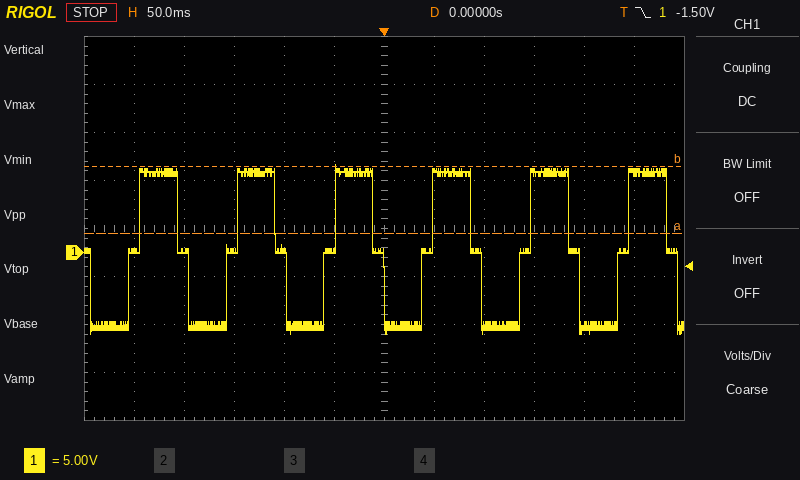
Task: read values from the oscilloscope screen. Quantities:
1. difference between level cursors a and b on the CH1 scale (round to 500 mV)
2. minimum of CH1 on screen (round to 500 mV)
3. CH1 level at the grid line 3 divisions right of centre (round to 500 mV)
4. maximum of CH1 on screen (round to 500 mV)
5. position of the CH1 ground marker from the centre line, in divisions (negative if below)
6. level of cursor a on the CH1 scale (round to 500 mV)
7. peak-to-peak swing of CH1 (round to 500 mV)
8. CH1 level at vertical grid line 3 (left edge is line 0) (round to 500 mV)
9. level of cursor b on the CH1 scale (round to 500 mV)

7.0 V
-8.5 V
8.5 V
9.0 V
-0.5 div
2.0 V
17.5 V
0.0 V
9.0 V
